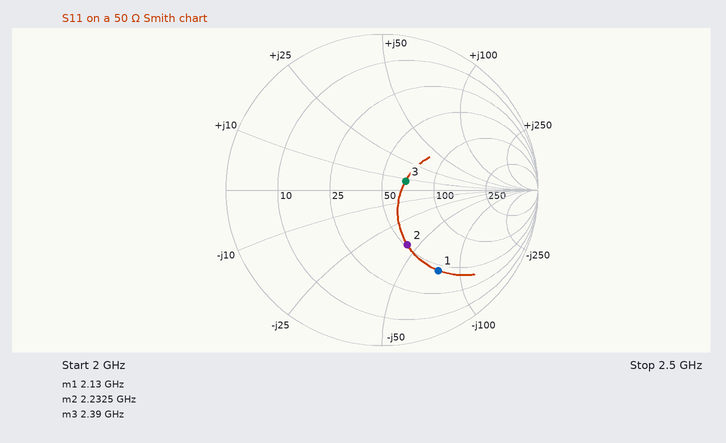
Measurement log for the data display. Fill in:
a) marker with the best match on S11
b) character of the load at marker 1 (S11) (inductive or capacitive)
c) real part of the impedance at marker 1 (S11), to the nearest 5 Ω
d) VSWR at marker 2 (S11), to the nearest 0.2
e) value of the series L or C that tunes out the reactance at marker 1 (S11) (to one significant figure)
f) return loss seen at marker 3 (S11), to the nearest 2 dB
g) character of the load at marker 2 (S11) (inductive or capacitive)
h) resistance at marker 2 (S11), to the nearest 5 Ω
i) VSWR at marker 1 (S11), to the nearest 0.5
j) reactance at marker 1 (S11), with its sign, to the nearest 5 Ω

marker 3
capacitive
45 Ω
2.2
6 nH
16 dB
capacitive
50 Ω
4.5
-75 Ω
